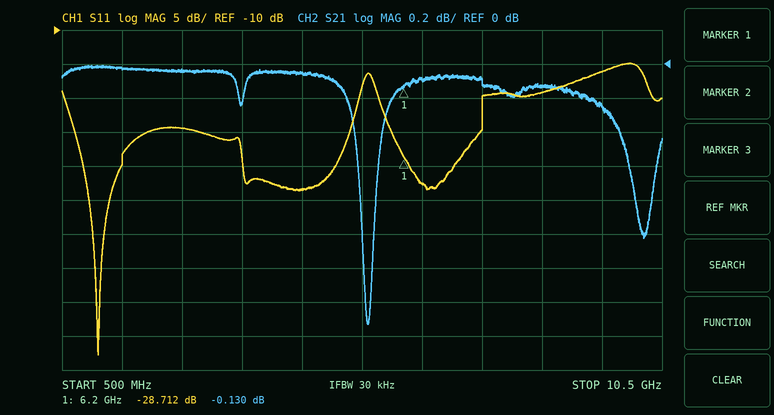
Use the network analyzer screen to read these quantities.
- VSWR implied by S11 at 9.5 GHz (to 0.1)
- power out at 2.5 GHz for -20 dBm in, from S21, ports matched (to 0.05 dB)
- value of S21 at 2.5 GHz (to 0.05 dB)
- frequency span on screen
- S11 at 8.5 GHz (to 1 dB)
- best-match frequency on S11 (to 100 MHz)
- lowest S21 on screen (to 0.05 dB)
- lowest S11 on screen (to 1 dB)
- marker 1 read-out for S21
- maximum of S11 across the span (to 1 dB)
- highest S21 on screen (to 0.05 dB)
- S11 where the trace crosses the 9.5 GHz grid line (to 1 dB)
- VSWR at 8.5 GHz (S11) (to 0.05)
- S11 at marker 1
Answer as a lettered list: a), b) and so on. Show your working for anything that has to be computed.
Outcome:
a) |Γ| = 10^(-16/20) = 0.1585; VSWR = (1 + 0.1585)/(1 − 0.1585) ≈ 1.4
b) -20 dBm + (-0.05 dB) = -20.05 dBm
c) -0.05 dB
d) 10 GHz
e) -19 dB
f) 1.1 GHz
g) -1.55 dB
h) -58 dB
i) -0.130 dB
j) -15 dB
k) 0.00 dB
l) -16 dB
m) |Γ| = 10^(-19/20) = 0.1122; VSWR = (1 + 0.1122)/(1 − 0.1122) ≈ 1.25
n) -28.712 dB
